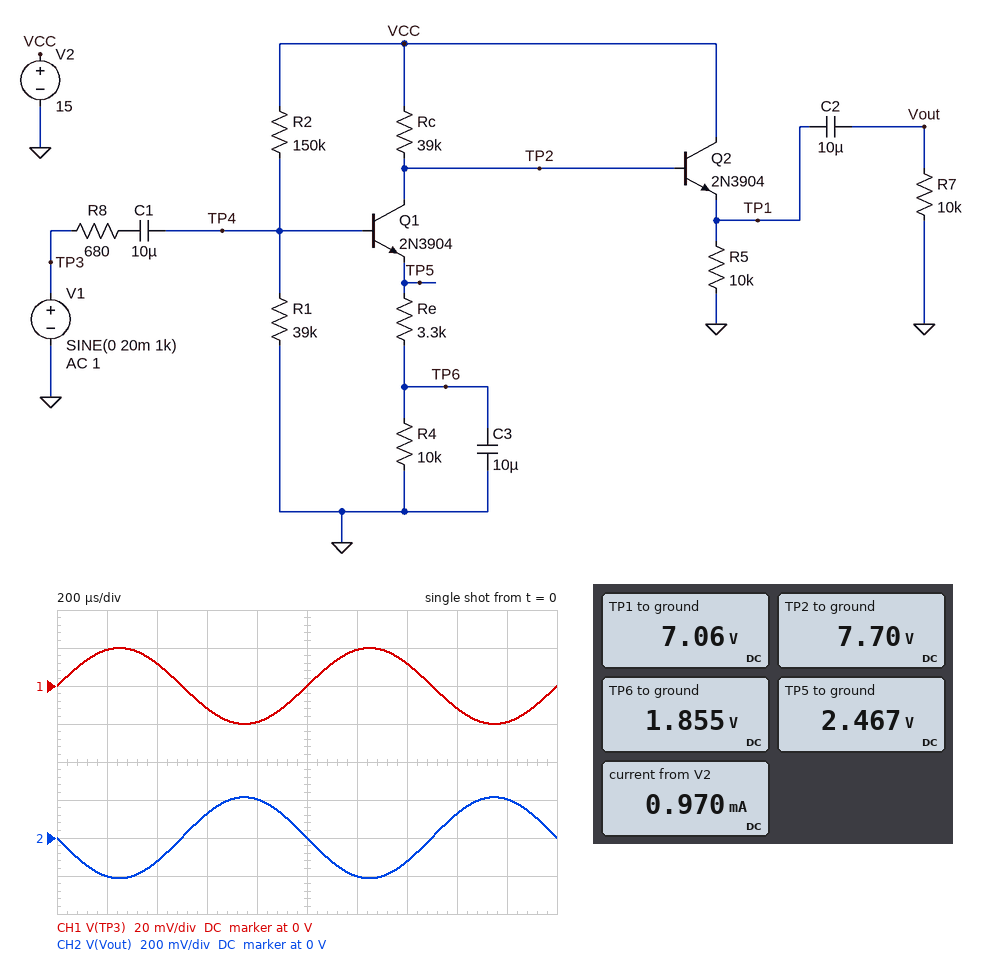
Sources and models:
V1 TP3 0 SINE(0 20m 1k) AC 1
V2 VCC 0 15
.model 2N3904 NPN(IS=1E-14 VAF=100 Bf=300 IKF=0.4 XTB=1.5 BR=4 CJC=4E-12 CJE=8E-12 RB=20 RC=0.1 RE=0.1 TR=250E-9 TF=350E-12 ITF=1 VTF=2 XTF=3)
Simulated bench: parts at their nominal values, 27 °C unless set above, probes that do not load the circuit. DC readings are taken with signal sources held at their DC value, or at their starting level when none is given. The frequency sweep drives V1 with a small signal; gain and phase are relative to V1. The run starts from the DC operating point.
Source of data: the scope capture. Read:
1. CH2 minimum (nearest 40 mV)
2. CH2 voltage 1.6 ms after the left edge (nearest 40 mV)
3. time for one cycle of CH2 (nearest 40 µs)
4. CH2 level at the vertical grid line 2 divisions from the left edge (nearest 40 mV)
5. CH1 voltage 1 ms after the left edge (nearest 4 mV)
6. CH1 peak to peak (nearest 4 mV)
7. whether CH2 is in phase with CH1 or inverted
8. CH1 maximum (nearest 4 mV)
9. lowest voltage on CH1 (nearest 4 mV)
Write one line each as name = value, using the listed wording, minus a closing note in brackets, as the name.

CH2 minimum = -200 mV
CH2 voltage 1.6 ms after the left edge = 120 mV
time for one cycle of CH2 = 1.00 ms
CH2 level at the vertical grid line 2 divisions from the left edge = -120 mV
CH1 voltage 1 ms after the left edge = 0 V
CH1 peak to peak = 40 mV
whether CH2 is in phase with CH1 or inverted = inverted
CH1 maximum = 20 mV
lowest voltage on CH1 = -20 mV
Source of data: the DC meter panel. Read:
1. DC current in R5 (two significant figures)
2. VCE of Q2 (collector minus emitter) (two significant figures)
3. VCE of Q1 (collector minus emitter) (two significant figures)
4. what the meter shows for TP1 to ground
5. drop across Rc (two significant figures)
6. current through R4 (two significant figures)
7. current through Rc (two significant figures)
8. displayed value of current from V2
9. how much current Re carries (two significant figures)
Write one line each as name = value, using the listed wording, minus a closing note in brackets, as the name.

DC current in R5 = 710 µA
VCE of Q2 (collector minus emitter) = 7.9 V
VCE of Q1 (collector minus emitter) = 5.2 V
what the meter shows for TP1 to ground = 7.06 V
drop across Rc = 7.3 V
current through R4 = 190 µA
current through Rc = 190 µA
displayed value of current from V2 = 0.970 mA
how much current Re carries = 190 µA
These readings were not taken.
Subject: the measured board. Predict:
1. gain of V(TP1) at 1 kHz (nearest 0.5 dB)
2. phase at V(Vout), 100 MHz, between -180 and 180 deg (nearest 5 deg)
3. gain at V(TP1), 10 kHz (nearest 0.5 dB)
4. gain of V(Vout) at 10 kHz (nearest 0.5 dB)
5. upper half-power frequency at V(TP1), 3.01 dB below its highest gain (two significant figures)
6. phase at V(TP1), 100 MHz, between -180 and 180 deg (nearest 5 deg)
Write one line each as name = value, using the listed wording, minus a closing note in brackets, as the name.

gain of V(TP1) at 1 kHz = 20.5 dB
phase at V(Vout), 100 MHz, between -180 and 180 deg = -15 deg
gain at V(TP1), 10 kHz = 20.5 dB
gain of V(Vout) at 10 kHz = 20.5 dB
upper half-power frequency at V(TP1), 3.01 dB below its highest gain = 930 kHz
phase at V(TP1), 100 MHz, between -180 and 180 deg = -15 deg
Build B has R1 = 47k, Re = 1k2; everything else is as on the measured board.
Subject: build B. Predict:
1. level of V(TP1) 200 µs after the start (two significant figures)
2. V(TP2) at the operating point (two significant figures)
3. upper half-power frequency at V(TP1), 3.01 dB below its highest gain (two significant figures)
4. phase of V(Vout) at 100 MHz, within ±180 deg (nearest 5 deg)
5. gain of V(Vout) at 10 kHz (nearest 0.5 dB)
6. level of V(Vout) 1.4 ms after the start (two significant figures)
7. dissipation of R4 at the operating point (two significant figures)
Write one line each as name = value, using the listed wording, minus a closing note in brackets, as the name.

level of V(TP1) 200 µs after the start = 3.6 V
V(TP2) at the operating point = 4.8 V
upper half-power frequency at V(TP1), 3.01 dB below its highest gain = 660 kHz
phase of V(Vout) at 100 MHz, within ±180 deg = -10 deg
gain of V(Vout) at 10 kHz = 29.0 dB
level of V(Vout) 1.4 ms after the start = -320 mV
dissipation of R4 at the operating point = 680 µW
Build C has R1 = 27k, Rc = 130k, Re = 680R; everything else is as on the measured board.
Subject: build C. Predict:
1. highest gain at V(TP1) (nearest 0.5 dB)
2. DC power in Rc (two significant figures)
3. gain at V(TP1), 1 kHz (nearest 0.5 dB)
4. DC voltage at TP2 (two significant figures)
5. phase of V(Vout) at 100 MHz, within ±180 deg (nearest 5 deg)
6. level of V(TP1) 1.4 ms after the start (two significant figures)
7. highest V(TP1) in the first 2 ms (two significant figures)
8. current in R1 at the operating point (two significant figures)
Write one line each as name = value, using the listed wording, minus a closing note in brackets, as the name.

highest gain at V(TP1) = -6.0 dB
DC power in Rc = 1.4 mW
gain at V(TP1), 1 kHz = -20.0 dB
DC voltage at TP2 = 1.3 V
phase of V(Vout) at 100 MHz, within ±180 deg = -20 deg
level of V(TP1) 1.4 ms after the start = 740 mV
highest V(TP1) in the first 2 ms = 750 mV
current in R1 at the operating point = 71 µA
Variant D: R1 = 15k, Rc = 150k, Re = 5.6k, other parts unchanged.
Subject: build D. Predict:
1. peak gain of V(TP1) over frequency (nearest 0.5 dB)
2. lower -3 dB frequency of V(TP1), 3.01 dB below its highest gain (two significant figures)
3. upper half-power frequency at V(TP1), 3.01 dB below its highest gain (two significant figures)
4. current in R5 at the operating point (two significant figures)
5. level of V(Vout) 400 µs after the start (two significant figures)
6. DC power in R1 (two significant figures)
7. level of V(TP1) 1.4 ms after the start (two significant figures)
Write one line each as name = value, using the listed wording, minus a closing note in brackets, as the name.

peak gain of V(TP1) over frequency = 26.5 dB
lower -3 dB frequency of V(TP1), 3.01 dB below its highest gain = 3.8 Hz
upper half-power frequency at V(TP1), 3.01 dB below its highest gain = 280 kHz
current in R5 at the operating point = 650 µA
level of V(Vout) 400 µs after the start = -240 mV
DC power in R1 = 120 µW
level of V(TP1) 1.4 ms after the start = 6.3 V
